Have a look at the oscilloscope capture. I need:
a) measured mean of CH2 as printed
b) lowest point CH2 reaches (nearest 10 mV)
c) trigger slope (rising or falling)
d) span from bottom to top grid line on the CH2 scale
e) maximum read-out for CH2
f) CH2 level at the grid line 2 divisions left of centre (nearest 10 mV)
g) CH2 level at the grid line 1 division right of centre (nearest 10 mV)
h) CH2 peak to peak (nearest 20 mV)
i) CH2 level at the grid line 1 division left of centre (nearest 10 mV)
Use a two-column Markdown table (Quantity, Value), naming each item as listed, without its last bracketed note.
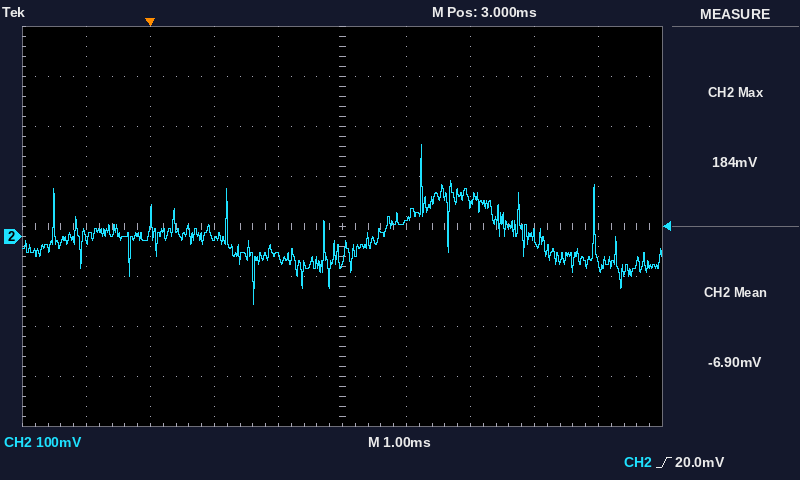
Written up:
| Quantity | Value |
|---|---|
| measured mean of CH2 as printed | -6.90 mV |
| lowest point CH2 reaches | -140 mV |
| trigger slope | rising |
| span from bottom to top grid line on the CH2 scale | 800 mV |
| maximum read-out for CH2 | 184 mV |
| CH2 level at the grid line 2 divisions left of centre | 0 mV |
| CH2 level at the grid line 1 division right of centre | 30 mV |
| CH2 peak to peak | 320 mV |
| CH2 level at the grid line 1 division left of centre | -40 mV |
